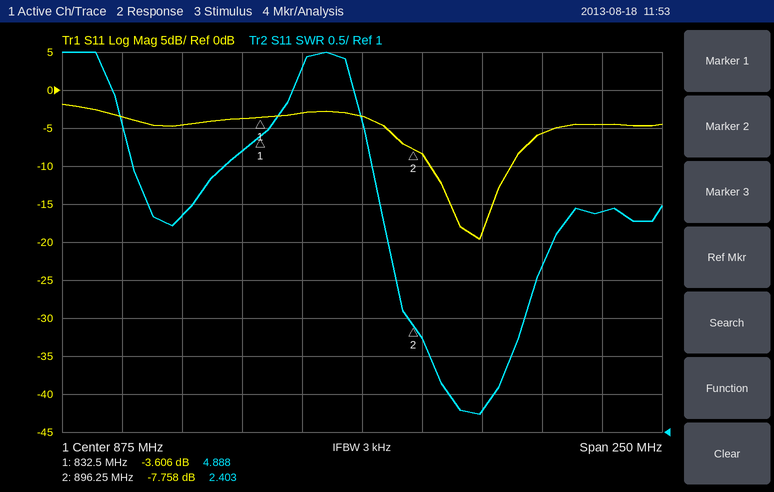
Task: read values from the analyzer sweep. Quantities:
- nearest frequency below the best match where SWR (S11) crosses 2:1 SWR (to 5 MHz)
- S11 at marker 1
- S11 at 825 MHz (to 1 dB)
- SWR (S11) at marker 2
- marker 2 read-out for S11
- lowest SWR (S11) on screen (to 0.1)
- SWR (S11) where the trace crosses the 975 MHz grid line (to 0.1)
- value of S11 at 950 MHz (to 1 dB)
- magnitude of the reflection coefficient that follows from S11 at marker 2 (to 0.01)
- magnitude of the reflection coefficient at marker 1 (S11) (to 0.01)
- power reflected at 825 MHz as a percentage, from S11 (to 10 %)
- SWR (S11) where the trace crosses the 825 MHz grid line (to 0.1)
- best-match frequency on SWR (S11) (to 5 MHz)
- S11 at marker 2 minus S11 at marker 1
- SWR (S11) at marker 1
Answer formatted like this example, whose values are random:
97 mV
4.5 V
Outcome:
905 MHz
-3.606 dB
-4 dB
2.403
-7.758 dB
1.2
3.9
-6 dB
0.41
0.66
40 %
4.7
925 MHz
-4.152 dB
4.888
